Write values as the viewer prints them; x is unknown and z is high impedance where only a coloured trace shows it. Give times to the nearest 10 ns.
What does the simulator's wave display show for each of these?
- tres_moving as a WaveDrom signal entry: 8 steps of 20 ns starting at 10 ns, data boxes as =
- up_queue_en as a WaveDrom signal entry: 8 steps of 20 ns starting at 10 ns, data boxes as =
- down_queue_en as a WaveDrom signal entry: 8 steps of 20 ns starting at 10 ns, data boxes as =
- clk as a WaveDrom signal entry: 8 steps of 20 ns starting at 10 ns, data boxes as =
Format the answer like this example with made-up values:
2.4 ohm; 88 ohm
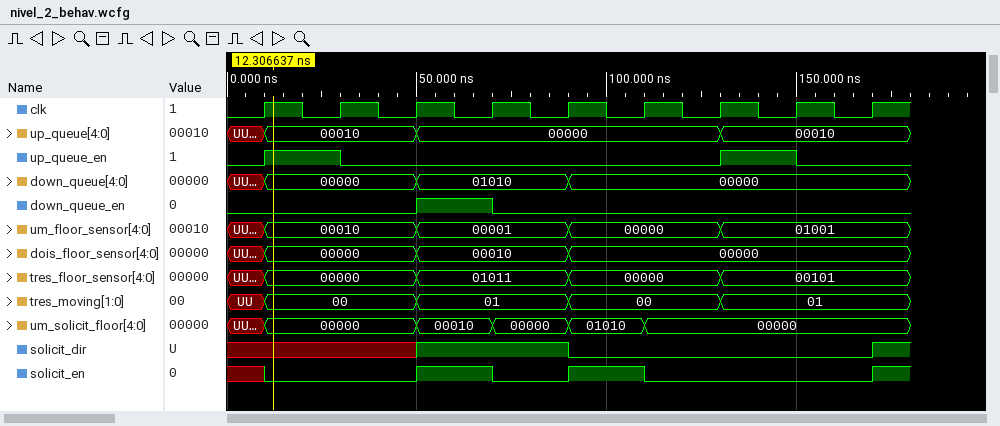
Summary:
{name: 'tres_moving', wave: '=.=.=.=.', data: '00 01 00 01'}; {name: 'up_queue_en', wave: '10....10'}; {name: 'down_queue_en', wave: '0.10....'}; {name: 'clk', wave: 'p.......'}
